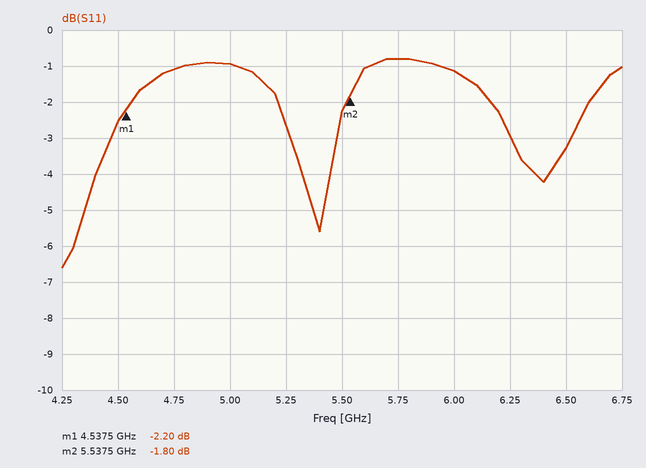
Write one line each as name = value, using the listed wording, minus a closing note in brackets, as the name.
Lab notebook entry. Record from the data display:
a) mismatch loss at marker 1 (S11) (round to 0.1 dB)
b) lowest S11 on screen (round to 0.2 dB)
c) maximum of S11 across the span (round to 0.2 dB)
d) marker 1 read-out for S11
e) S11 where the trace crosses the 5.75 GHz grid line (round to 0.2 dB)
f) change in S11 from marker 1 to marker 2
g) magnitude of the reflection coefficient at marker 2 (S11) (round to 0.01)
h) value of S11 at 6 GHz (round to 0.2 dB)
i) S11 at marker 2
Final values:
mismatch loss at marker 1 (S11) = 4.0 dB
lowest S11 on screen = -6.6 dB
maximum of S11 across the span = -0.8 dB
marker 1 read-out for S11 = -2.20 dB
S11 where the trace crosses the 5.75 GHz grid line = -0.8 dB
change in S11 from marker 1 to marker 2 = 0.40 dB
magnitude of the reflection coefficient at marker 2 (S11) = 0.81
value of S11 at 6 GHz = -1.2 dB
S11 at marker 2 = -1.80 dB
